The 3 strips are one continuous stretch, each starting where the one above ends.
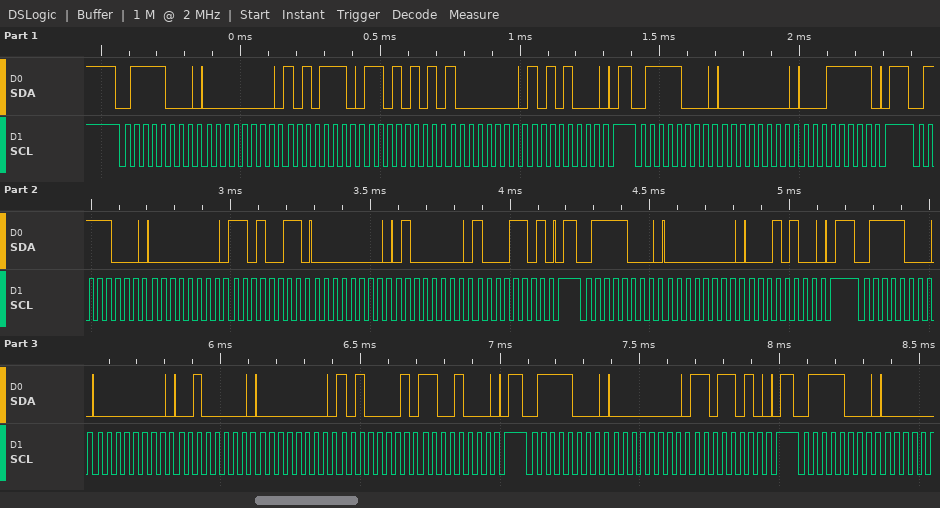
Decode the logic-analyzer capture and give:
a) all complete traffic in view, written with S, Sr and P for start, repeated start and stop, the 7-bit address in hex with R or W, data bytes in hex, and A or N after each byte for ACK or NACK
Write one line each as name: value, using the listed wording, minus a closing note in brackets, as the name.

all complete traffic in view, written with S, Sr and P for start, repeated start and stop, the 7-bit address in hex with R or W, data bytes in hex, and A or N after each byte for ACK or NACK: S 3CW A 00 A AE A D5 A 80 A A8 A P S 3CW A 00 A 1F A P S 3CW A 00 A D3 A 00 A 40 A 8D A P S 3CW A 00 A 14 A P S 3CW A 00 A 20 A 00 A A1 A C8 A P S 3CW A 00 A DA A P S 3CW A
